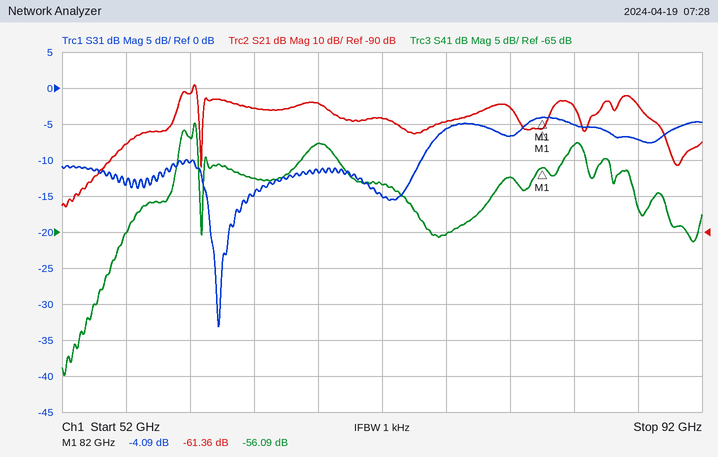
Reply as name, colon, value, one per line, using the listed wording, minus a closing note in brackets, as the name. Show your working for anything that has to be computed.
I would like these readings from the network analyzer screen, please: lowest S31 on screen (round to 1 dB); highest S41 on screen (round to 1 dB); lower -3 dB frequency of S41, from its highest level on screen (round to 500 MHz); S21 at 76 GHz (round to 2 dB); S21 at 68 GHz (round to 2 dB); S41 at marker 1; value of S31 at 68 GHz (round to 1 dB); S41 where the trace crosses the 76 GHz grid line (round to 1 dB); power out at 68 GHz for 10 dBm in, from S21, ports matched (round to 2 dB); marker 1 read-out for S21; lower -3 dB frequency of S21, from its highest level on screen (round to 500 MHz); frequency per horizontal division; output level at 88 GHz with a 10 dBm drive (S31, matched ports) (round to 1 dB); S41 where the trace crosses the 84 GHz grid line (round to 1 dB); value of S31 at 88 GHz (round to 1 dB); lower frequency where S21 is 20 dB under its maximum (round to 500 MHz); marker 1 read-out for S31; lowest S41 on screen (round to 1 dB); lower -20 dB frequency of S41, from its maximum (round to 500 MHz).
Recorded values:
lowest S31 on screen: -33 dB
highest S41 on screen: -50 dB
lower -3 dB frequency of S41, from its highest level on screen: 59.5 GHz
S21 at 76 GHz: -60 dB
S21 at 68 GHz: -54 dB
S41 at marker 1: -56.09 dB
value of S31 at 68 GHz: -12 dB
S41 where the trace crosses the 76 GHz grid line: -65 dB
power out at 68 GHz for 10 dBm in, from S21, ports matched: 10 dBm + (-54 dB) = -44 dBm
marker 1 read-out for S21: -61.36 dB
lower -3 dB frequency of S21, from its highest level on screen: 59.5 GHz
frequency per horizontal division: 4 GHz
output level at 88 GHz with a 10 dBm drive (S31, matched ports): 10 dBm + (-7 dB) = 3 dBm
S41 where the trace crosses the 84 GHz grid line: -53 dB
value of S31 at 88 GHz: -7 dB
lower frequency where S21 is 20 dB under its maximum: 55.0 GHz
marker 1 read-out for S31: -4.09 dB
lowest S41 on screen: -85 dB
lower -20 dB frequency of S41, from its maximum: 55.0 GHz
